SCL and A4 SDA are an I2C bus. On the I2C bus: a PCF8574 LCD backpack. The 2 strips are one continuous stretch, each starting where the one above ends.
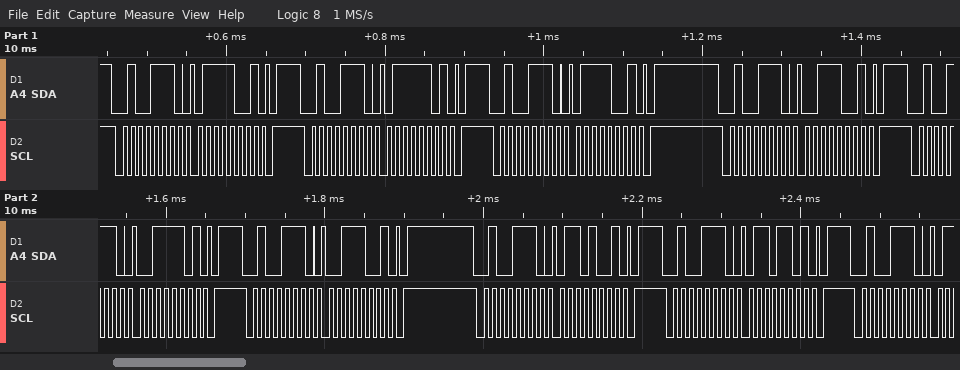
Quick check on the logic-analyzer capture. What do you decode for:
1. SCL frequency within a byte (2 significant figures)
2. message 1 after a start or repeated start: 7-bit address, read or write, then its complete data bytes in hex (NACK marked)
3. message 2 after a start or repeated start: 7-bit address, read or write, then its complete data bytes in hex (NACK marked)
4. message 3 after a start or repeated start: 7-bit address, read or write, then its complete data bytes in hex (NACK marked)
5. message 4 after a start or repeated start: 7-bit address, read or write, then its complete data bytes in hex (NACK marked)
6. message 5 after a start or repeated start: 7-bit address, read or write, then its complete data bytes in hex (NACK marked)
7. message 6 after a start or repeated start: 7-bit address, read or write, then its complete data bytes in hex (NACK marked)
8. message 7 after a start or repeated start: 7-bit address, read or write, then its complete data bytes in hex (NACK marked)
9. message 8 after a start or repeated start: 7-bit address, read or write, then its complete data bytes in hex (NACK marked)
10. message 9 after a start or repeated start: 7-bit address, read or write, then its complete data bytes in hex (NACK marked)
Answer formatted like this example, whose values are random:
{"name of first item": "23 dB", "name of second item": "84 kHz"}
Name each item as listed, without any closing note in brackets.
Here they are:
{"SCL frequency within a byte": "100 kHz", "message 1 after a start or repeated start: 7-bit address, read or write, then its complete data bytes in hex": "0x27 write: 79", "message 2 after a start or repeated start: 7-bit address, read or write, then its complete data bytes in hex": "0x27 write: 7D", "message 3 after a start or repeated start: 7-bit address, read or write, then its complete data bytes in hex": "0x27 write: 79", "message 4 after a start or repeated start: 7-bit address, read or write, then its complete data bytes in hex": "0x27 write: 39", "message 5 after a start or repeated start: 7-bit address, read or write, then its complete data bytes in hex": "0x27 write: 3D", "message 6 after a start or repeated start: 7-bit address, read or write, then its complete data bytes in hex": "0x27 write: 39", "message 7 after a start or repeated start: 7-bit address, read or write, then its complete data bytes in hex": "0x27 write: 69", "message 8 after a start or repeated start: 7-bit address, read or write, then its complete data bytes in hex": "0x27 write: 6D", "message 9 after a start or repeated start: 7-bit address, read or write, then its complete data bytes in hex": "0x27 write"}
